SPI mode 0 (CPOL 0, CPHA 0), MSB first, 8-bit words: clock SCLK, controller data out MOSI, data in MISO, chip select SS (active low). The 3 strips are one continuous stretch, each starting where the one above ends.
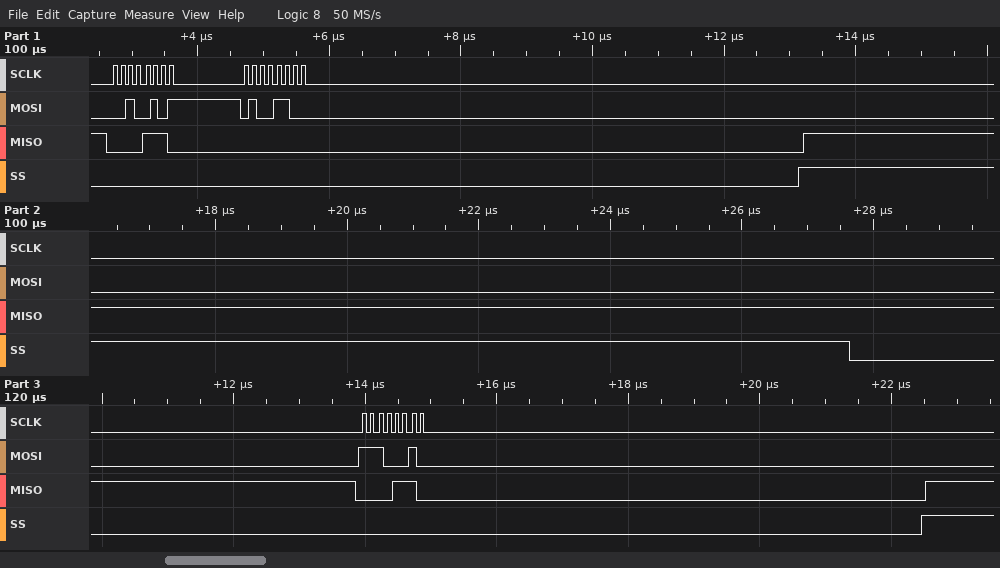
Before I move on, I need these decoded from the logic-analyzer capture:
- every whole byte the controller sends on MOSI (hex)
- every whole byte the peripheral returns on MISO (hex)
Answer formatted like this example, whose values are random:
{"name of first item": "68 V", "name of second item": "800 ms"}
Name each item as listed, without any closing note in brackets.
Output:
{"every whole byte the controller sends on MOSI": "0x25 0x4C 0xE2", "every whole byte the peripheral returns on MISO": "0x0E 0x00 0x0E"}
